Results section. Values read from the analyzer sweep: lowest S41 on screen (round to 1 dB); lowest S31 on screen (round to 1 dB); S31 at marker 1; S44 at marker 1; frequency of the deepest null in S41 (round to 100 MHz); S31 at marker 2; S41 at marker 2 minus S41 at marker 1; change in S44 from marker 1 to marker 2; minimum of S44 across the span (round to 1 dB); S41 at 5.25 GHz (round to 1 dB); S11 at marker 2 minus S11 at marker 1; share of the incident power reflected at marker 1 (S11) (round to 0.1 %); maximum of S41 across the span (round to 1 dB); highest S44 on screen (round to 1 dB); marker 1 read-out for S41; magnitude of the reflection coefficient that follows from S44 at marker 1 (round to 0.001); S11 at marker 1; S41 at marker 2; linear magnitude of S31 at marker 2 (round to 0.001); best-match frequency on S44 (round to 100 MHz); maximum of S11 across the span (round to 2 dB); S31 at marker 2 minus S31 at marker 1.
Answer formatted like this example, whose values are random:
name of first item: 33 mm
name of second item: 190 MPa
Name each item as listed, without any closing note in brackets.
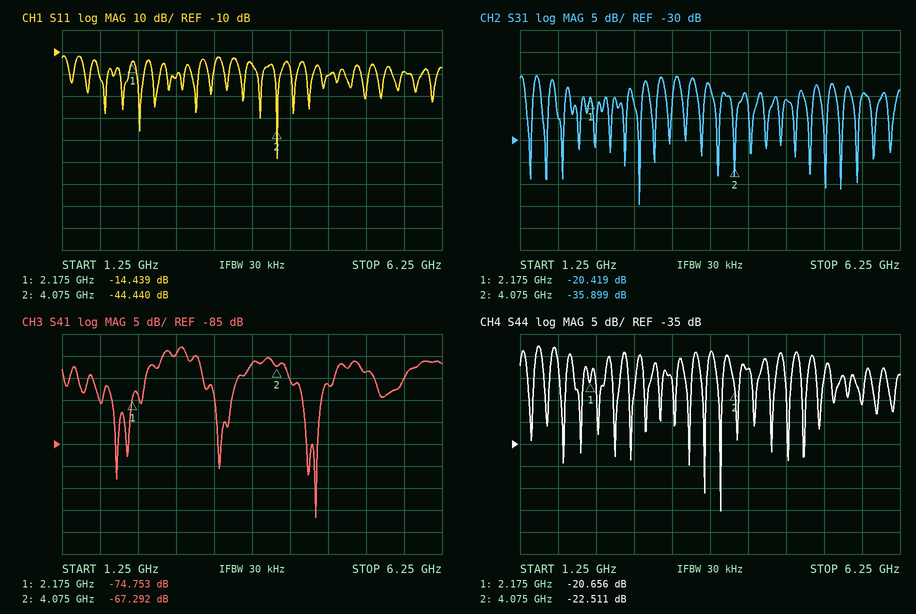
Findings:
lowest S41 on screen: -102 dB
lowest S31 on screen: -45 dB
S31 at marker 1: -20.419 dB
S44 at marker 1: -20.656 dB
frequency of the deepest null in S41: 4.6 GHz
S31 at marker 2: -35.899 dB
S41 at marker 2 minus S41 at marker 1: 7.461 dB
change in S44 from marker 1 to marker 2: -1.855 dB
minimum of S44 across the span: -50 dB
S41 at 5.25 GHz: -69 dB
S11 at marker 2 minus S11 at marker 1: -30.001 dB
share of the incident power reflected at marker 1 (S11): 3.6 %
maximum of S41 across the span: -63 dB
highest S44 on screen: -13 dB
marker 1 read-out for S41: -74.753 dB
magnitude of the reflection coefficient that follows from S44 at marker 1: 0.093
S11 at marker 1: -14.439 dB
S41 at marker 2: -67.292 dB
linear magnitude of S31 at marker 2: 0.016
best-match frequency on S44: 3.9 GHz
maximum of S11 across the span: -12 dB
S31 at marker 2 minus S31 at marker 1: -15.480 dB
